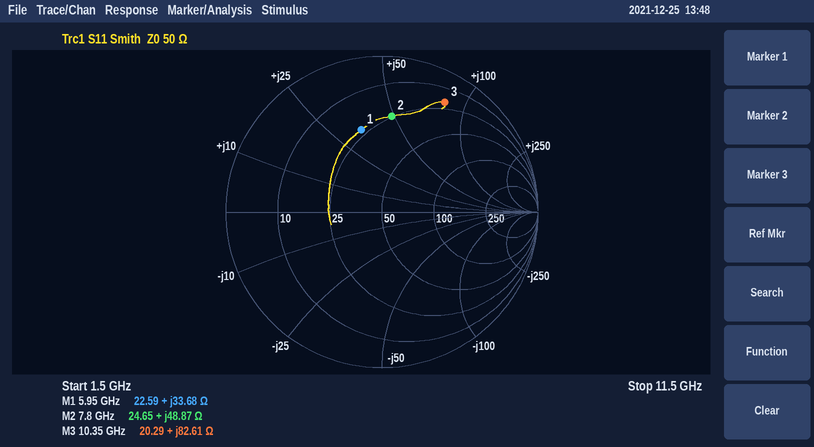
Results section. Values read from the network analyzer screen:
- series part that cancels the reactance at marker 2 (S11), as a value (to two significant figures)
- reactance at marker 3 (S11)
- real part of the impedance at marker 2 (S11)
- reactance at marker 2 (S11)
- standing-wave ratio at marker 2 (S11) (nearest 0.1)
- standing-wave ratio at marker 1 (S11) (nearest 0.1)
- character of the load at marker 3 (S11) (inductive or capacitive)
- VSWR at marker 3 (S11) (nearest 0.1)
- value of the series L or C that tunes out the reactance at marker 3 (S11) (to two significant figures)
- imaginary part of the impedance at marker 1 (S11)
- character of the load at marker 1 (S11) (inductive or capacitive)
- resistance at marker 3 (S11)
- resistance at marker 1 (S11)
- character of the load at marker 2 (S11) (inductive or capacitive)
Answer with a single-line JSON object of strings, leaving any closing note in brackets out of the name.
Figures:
{"series part that cancels the reactance at marker 2 (S11), as a value": "420 fF", "reactance at marker 3": "+82.61 Ω", "real part of the impedance at marker 2": "24.65 Ω", "reactance at marker 2": "+48.87 Ω", "standing-wave ratio at marker 2 (S11)": "4.2", "standing-wave ratio at marker 1 (S11)": "3.4", "character of the load at marker 3 (S11)": "inductive", "VSWR at marker 3 (S11)": "9.5", "value of the series L or C that tunes out the reactance at marker 3 (S11)": "190 fF", "imaginary part of the impedance at marker 1": "+33.68 Ω", "character of the load at marker 1 (S11)": "inductive", "resistance at marker 3": "20.29 Ω", "resistance at marker 1": "22.59 Ω", "character of the load at marker 2 (S11)": "inductive"}
